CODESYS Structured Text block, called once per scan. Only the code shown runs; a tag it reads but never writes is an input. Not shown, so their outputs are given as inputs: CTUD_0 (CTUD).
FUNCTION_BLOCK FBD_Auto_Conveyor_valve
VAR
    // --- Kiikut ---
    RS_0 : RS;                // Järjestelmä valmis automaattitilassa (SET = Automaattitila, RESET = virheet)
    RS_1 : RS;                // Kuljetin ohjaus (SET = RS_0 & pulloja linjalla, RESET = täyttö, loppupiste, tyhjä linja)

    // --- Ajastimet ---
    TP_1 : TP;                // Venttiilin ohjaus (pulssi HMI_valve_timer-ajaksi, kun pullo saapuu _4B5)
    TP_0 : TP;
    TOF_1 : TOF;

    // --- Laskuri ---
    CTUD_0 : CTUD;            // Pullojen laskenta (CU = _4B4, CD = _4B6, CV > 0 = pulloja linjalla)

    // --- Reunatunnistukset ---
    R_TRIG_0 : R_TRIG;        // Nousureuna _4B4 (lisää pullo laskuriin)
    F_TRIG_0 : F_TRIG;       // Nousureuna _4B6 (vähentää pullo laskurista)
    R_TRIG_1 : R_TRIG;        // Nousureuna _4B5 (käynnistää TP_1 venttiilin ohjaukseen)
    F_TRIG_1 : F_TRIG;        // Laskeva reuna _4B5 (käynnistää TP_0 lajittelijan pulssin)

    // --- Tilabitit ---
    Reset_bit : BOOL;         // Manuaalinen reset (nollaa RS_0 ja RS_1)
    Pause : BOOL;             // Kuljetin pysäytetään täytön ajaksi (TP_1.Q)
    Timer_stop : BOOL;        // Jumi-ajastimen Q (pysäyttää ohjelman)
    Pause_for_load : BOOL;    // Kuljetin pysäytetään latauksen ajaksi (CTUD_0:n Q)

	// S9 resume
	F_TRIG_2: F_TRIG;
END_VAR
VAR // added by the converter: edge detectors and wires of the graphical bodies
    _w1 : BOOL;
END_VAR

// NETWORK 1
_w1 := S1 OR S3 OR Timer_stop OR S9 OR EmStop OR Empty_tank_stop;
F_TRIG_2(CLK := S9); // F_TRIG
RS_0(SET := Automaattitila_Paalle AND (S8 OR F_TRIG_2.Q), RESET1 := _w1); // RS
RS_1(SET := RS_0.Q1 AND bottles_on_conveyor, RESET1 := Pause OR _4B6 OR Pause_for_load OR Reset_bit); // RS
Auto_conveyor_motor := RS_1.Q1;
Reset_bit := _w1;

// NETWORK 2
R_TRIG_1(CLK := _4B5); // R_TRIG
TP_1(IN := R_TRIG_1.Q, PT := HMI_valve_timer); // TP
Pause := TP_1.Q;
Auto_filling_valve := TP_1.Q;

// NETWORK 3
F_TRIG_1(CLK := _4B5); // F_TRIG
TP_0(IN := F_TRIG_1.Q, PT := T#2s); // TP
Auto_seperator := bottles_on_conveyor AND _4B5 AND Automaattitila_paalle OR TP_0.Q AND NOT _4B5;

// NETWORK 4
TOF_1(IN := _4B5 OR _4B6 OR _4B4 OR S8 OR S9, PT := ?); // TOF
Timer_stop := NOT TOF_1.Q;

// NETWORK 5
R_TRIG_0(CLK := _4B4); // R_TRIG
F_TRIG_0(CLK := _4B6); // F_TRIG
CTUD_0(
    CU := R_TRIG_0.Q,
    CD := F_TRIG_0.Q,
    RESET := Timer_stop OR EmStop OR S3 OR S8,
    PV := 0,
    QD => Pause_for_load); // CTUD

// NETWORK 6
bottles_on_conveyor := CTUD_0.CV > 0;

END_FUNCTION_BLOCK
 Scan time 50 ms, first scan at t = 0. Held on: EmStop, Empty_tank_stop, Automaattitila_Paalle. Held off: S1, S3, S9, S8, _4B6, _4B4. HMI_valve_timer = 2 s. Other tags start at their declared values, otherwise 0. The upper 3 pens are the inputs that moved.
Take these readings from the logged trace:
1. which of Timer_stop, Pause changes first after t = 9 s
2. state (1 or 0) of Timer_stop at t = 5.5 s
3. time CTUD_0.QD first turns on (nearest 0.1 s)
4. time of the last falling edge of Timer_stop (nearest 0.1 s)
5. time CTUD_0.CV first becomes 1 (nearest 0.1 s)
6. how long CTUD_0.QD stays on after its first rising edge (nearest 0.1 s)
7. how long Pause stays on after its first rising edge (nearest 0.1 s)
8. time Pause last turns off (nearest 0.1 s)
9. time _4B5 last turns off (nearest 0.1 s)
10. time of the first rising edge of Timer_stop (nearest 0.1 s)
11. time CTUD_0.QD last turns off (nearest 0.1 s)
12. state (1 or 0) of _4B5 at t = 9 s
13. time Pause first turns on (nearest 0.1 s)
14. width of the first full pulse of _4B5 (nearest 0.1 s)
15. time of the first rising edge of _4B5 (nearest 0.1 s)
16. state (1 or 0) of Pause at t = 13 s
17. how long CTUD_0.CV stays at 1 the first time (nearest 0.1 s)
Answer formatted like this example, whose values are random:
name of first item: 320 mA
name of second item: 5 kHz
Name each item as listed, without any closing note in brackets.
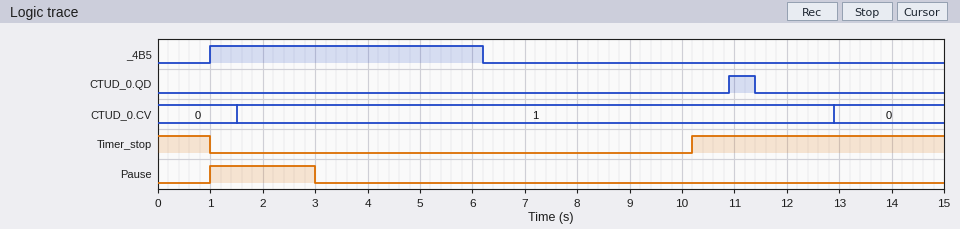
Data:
which of Timer_stop, Pause changes first after t = 9 s: Timer_stop
state (1 or 0) of Timer_stop at t = 5.5 s: 0
time CTUD_0.QD first turns on: 10.9 s
time of the last falling edge of Timer_stop: 1.0 s
time CTUD_0.CV first becomes 1: 1.5 s
how long CTUD_0.QD stays on after its first rising edge: 0.5 s
how long Pause stays on after its first rising edge: 2.0 s
time Pause last turns off: 3.0 s
time _4B5 last turns off: 6.2 s
time of the first rising edge of Timer_stop: 10.2 s
time CTUD_0.QD last turns off: 11.4 s
state (1 or 0) of _4B5 at t = 9 s: 0
time Pause first turns on: 1.0 s
width of the first full pulse of _4B5: 5.2 s
time of the first rising edge of _4B5: 1.0 s
state (1 or 0) of Pause at t = 13 s: 0
how long CTUD_0.CV stays at 1 the first time: 11.4 s
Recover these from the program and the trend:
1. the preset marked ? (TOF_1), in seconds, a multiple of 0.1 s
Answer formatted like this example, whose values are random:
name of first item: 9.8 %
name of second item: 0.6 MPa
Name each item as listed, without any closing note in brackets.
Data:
the preset marked ? (TOF_1), in seconds, a multiple of 0.1 s: 4.0 s
